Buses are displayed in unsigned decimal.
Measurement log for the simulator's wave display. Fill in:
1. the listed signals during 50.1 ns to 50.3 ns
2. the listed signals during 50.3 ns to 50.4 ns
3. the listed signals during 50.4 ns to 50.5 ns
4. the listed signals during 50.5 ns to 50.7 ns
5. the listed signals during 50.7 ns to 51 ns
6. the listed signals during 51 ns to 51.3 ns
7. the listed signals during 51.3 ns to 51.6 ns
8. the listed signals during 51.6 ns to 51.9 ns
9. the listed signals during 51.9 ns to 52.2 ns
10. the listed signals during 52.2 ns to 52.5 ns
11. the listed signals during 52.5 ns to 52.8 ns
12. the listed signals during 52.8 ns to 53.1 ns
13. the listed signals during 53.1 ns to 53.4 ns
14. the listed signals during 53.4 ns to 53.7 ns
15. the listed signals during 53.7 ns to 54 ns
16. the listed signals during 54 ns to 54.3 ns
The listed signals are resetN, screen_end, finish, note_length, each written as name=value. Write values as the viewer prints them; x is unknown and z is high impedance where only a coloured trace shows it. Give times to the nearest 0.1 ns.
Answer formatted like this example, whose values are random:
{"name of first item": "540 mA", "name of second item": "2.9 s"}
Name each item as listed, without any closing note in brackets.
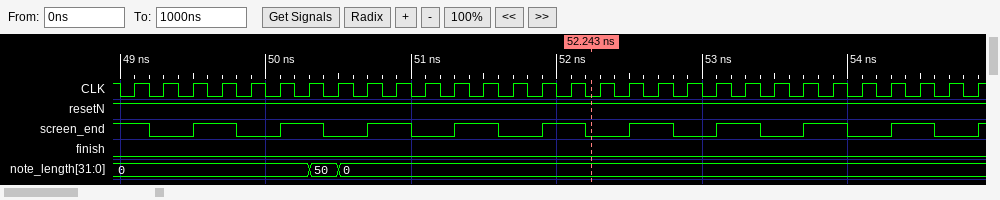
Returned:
{"the listed signals during 50.1 ns to 50.3 ns": "resetN=1, screen_end=1, finish=0, note_length=0", "the listed signals during 50.3 ns to 50.4 ns": "resetN=1, screen_end=1, finish=0, note_length=50", "the listed signals during 50.4 ns to 50.5 ns": "resetN=1, screen_end=0, finish=0, note_length=50", "the listed signals during 50.5 ns to 50.7 ns": "resetN=1, screen_end=0, finish=0, note_length=0", "the listed signals during 50.7 ns to 51 ns": "resetN=1, screen_end=1, finish=0, note_length=0", "the listed signals during 51 ns to 51.3 ns": "resetN=1, screen_end=0, finish=0, note_length=0", "the listed signals during 51.3 ns to 51.6 ns": "resetN=1, screen_end=1, finish=0, note_length=0", "the listed signals during 51.6 ns to 51.9 ns": "resetN=1, screen_end=0, finish=0, note_length=0", "the listed signals during 51.9 ns to 52.2 ns": "resetN=1, screen_end=1, finish=0, note_length=0", "the listed signals during 52.2 ns to 52.5 ns": "resetN=1, screen_end=0, finish=0, note_length=0", "the listed signals during 52.5 ns to 52.8 ns": "resetN=1, screen_end=1, finish=0, note_length=0", "the listed signals during 52.8 ns to 53.1 ns": "resetN=1, screen_end=0, finish=0, note_length=0", "the listed signals during 53.1 ns to 53.4 ns": "resetN=1, screen_end=1, finish=0, note_length=0", "the listed signals during 53.4 ns to 53.7 ns": "resetN=1, screen_end=0, finish=0, note_length=0", "the listed signals during 53.7 ns to 54 ns": "resetN=1, screen_end=1, finish=0, note_length=0", "the listed signals during 54 ns to 54.3 ns": "resetN=1, screen_end=0, finish=0, note_length=0"}
